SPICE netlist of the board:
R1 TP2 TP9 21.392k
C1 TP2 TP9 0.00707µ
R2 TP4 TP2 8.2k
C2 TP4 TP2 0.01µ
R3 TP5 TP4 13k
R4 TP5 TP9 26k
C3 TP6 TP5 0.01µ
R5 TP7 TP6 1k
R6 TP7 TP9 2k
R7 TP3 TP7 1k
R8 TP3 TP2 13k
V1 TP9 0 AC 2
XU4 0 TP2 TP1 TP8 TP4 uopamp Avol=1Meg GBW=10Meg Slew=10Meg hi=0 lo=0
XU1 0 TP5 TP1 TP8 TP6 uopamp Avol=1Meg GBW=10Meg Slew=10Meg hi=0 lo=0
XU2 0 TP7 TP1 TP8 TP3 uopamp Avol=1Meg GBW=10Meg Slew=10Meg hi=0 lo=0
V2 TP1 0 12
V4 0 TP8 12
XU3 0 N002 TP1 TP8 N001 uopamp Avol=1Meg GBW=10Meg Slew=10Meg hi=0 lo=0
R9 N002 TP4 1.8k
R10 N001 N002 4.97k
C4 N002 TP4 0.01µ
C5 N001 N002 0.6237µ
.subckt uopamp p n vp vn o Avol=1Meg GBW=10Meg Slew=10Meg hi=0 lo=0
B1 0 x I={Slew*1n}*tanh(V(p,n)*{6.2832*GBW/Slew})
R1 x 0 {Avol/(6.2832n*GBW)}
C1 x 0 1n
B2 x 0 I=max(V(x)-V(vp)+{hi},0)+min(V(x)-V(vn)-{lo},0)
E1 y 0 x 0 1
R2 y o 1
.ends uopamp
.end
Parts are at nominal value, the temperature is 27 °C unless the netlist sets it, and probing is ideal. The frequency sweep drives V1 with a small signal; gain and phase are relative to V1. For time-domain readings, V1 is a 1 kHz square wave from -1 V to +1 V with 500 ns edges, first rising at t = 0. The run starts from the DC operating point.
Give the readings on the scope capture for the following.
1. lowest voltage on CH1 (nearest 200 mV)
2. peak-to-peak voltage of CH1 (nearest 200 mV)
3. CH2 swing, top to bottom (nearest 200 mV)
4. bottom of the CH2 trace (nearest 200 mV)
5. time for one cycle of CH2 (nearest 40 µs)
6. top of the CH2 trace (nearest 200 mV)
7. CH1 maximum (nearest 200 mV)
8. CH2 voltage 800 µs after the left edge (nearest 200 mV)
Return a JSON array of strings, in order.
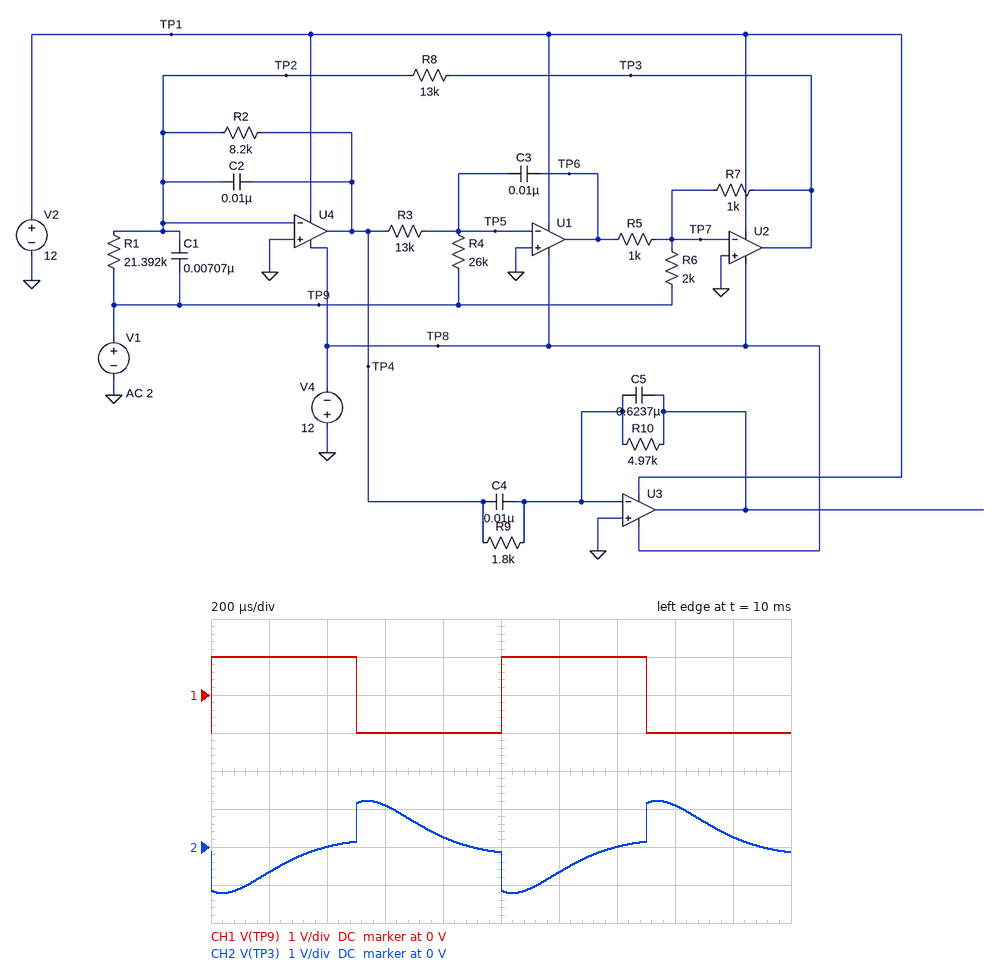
["-1.0 V", "2.0 V", "2.4 V", "-1.2 V", "1.00 ms", "1.2 V", "1.0 V", "200 mV"]
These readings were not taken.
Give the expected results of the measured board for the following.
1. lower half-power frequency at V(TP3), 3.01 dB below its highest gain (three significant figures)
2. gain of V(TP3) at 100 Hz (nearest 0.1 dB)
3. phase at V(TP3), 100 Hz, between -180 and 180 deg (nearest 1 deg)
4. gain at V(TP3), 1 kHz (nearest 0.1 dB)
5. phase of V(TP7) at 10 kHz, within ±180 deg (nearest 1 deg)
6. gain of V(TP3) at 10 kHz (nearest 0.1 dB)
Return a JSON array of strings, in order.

["622 Hz", "-13.8 dB", "-31 deg", "-2.8 dB", "87 deg", "-5.8 dB"]
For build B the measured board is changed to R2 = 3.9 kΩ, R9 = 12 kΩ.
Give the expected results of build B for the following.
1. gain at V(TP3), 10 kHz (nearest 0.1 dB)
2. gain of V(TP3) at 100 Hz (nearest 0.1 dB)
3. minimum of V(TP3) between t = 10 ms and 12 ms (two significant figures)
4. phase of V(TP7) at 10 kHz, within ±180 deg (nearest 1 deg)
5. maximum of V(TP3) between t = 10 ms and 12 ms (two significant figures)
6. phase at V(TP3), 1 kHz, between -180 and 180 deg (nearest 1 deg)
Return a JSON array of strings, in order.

["-5.5 dB", "0.4 dB", "-1.3 V", "88 deg", "1.3 V", "-131 deg"]
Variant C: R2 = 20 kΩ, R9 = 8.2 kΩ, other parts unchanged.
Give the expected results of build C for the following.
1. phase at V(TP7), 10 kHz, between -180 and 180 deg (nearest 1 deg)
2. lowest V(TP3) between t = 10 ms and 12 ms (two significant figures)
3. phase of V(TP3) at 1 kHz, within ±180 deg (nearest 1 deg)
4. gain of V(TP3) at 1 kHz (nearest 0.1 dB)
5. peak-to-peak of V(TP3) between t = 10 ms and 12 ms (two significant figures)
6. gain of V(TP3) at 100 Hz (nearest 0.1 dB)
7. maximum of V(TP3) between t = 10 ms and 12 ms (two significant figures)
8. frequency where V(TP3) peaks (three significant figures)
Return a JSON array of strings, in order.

["87 deg", "-1.1 V", "-141 deg", "-3.1 dB", "2.1 V", "-10.9 dB", "1.1 V", "1.31 kHz"]
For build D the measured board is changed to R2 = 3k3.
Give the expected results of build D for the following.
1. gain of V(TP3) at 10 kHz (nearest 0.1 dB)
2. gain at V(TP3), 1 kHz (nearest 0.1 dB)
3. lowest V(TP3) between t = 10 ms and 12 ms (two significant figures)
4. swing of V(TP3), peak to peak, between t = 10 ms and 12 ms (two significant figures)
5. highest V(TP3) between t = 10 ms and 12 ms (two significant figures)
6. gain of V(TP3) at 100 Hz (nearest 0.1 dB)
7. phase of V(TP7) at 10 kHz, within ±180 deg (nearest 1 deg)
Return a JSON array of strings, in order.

["-5.5 dB", "-2.4 dB", "-1.3 V", "2.7 V", "1.3 V", "2.4 dB", "89 deg"]
